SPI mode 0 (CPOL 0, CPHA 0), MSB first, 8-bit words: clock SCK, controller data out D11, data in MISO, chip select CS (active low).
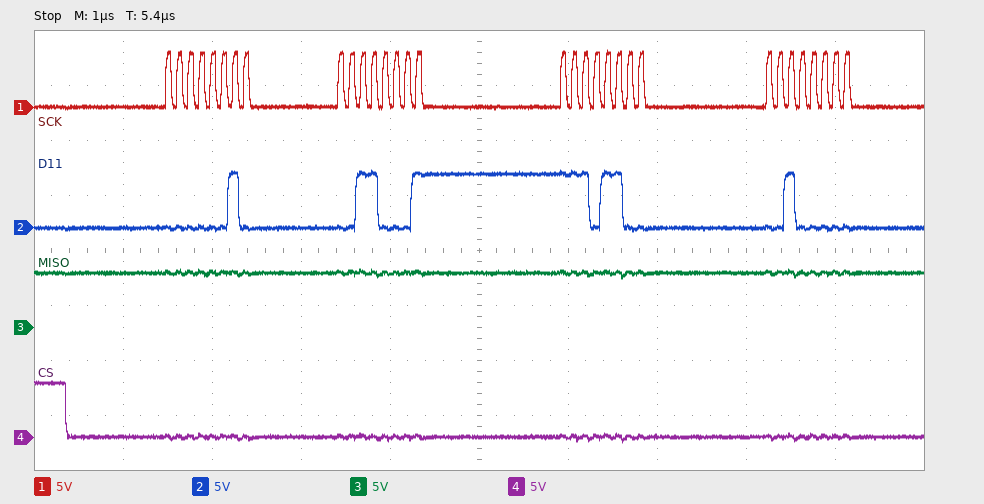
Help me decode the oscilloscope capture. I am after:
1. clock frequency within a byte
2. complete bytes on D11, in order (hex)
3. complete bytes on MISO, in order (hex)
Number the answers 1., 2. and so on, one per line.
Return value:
1. 8 MHz
2. 02 31 EC 20
3. FF FF FF FF
